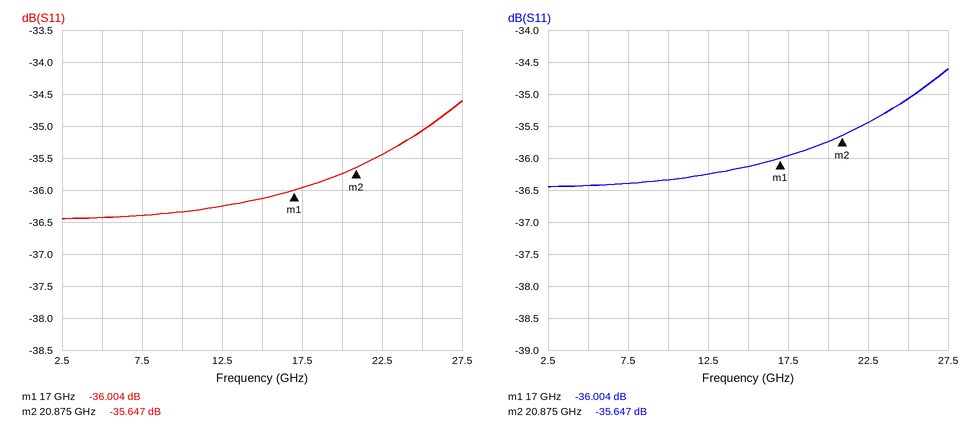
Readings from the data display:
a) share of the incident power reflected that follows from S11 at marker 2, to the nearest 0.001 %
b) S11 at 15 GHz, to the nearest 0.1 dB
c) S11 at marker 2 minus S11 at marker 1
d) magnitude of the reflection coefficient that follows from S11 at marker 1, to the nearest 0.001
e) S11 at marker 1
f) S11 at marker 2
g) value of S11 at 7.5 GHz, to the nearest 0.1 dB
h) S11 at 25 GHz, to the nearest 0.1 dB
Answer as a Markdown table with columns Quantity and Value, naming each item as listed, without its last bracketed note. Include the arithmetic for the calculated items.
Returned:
| Quantity | Value |
|---|---|
| share of the incident power reflected that follows from S11 at marker 2, to the nearest 0.001 % | 10^(-35.647/10) ≈ 0.027 % |
| S11 at 15 GHz, to the nearest 0.1 dB | -36.1 dB |
| S11 at marker 2 minus S11 at marker 1 | -35.647 − (-36.004) = 0.357 dB |
| magnitude of the reflection coefficient that follows from S11 at marker 1, to the nearest 0.001 | 10^(-36.004/20) ≈ 0.016 |
| S11 at marker 1 | -36.004 dB |
| S11 at marker 2 | -35.647 dB |
| value of S11 at 7.5 GHz, to the nearest 0.1 dB | -36.4 dB |
| S11 at 25 GHz, to the nearest 0.1 dB | -35.1 dB |
